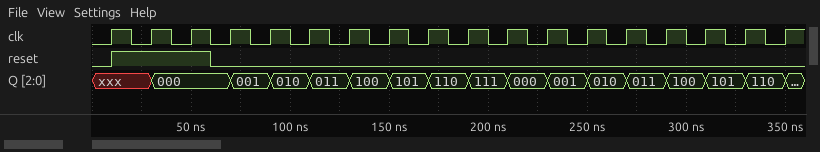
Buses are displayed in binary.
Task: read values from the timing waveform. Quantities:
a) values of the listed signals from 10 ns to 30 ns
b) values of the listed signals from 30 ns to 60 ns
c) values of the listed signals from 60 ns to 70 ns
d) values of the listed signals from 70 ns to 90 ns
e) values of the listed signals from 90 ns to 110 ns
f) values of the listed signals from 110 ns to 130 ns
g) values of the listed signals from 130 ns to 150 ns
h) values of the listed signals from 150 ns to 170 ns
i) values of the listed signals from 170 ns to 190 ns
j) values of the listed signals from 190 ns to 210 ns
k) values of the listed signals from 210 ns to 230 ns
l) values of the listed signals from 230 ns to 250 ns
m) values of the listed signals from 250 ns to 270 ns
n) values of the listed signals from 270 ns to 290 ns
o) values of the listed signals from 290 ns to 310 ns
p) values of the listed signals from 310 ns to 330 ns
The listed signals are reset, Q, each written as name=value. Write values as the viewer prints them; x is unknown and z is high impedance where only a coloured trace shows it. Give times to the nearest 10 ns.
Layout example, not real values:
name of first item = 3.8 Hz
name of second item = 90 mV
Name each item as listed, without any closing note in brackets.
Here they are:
values of the listed signals from 10 ns to 30 ns = reset=1, Q=xxx
values of the listed signals from 30 ns to 60 ns = reset=1, Q=000
values of the listed signals from 60 ns to 70 ns = reset=0, Q=000
values of the listed signals from 70 ns to 90 ns = reset=0, Q=001
values of the listed signals from 90 ns to 110 ns = reset=0, Q=010
values of the listed signals from 110 ns to 130 ns = reset=0, Q=011
values of the listed signals from 130 ns to 150 ns = reset=0, Q=100
values of the listed signals from 150 ns to 170 ns = reset=0, Q=101
values of the listed signals from 170 ns to 190 ns = reset=0, Q=110
values of the listed signals from 190 ns to 210 ns = reset=0, Q=111
values of the listed signals from 210 ns to 230 ns = reset=0, Q=000
values of the listed signals from 230 ns to 250 ns = reset=0, Q=001
values of the listed signals from 250 ns to 270 ns = reset=0, Q=010
values of the listed signals from 270 ns to 290 ns = reset=0, Q=011
values of the listed signals from 290 ns to 310 ns = reset=0, Q=100
values of the listed signals from 310 ns to 330 ns = reset=0, Q=101
